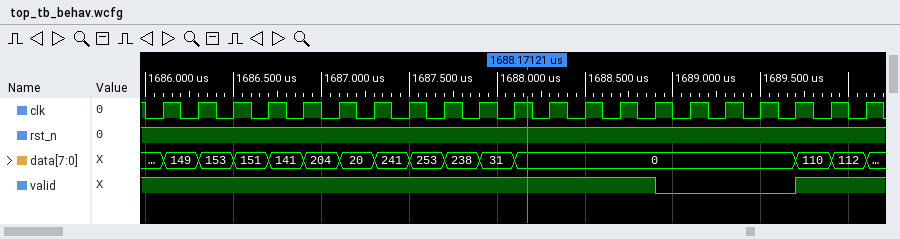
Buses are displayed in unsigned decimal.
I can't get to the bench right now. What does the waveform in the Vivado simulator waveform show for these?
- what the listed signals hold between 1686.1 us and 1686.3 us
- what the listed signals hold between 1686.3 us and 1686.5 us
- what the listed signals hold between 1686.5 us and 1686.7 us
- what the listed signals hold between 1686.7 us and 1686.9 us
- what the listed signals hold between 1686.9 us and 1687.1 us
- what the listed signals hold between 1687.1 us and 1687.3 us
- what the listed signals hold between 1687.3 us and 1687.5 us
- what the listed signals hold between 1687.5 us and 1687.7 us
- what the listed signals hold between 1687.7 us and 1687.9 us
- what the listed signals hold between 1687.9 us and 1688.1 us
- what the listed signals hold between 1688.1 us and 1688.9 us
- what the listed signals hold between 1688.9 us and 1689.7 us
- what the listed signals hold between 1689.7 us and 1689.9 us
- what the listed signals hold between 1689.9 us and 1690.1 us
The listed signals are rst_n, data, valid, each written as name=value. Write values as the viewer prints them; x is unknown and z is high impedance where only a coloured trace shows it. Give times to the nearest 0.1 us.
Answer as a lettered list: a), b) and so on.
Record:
a) rst_n=1, data=149, valid=1
b) rst_n=1, data=153, valid=1
c) rst_n=1, data=151, valid=1
d) rst_n=1, data=141, valid=1
e) rst_n=1, data=204, valid=1
f) rst_n=1, data=20, valid=1
g) rst_n=1, data=241, valid=1
h) rst_n=1, data=253, valid=1
i) rst_n=1, data=238, valid=1
j) rst_n=1, data=31, valid=1
k) rst_n=1, data=0, valid=1
l) rst_n=1, data=0, valid=0
m) rst_n=1, data=110, valid=1
n) rst_n=1, data=112, valid=1
